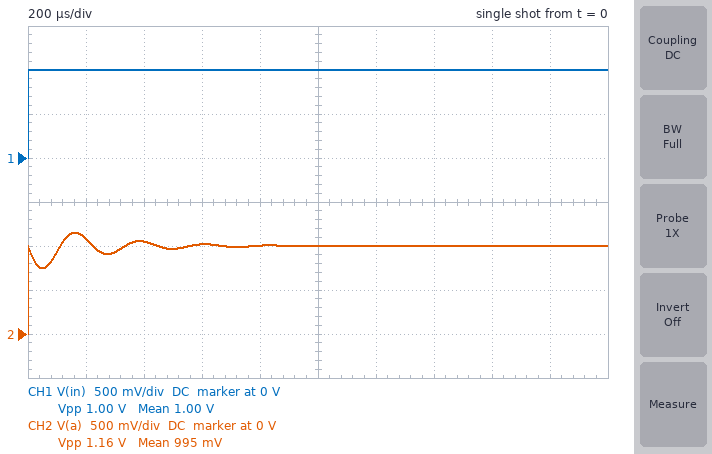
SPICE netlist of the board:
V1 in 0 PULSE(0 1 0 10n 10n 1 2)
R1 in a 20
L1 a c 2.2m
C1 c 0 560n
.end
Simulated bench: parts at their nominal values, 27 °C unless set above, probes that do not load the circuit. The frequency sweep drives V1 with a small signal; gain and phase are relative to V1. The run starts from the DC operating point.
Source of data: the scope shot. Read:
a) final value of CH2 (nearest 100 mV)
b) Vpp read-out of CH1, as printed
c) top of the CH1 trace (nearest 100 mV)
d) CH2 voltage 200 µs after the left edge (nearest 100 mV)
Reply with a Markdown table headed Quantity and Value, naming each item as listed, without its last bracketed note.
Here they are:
| Quantity | Value |
|---|---|
| final value of CH2 | 1.0 V |
| Vpp read-out of CH1, as printed | 1.00 V |
| top of the CH1 trace | 1.0 V |
| CH2 voltage 200 µs after the left edge | 1.1 V |
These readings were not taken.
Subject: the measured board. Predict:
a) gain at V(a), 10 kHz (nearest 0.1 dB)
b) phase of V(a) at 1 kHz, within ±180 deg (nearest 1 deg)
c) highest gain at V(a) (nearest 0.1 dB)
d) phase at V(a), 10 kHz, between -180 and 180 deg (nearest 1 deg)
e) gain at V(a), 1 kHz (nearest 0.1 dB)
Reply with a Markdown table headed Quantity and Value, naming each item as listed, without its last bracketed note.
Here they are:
| Quantity | Value |
|---|---|
| gain at V(a), 10 kHz | -0.1 dB |
| phase of V(a) at 1 kHz, within ±180 deg | -4 deg |
| highest gain at V(a) | 0 dB |
| phase at V(a), 10 kHz, between -180 and 180 deg | 10 deg |
| gain at V(a), 1 kHz | 0 dB |
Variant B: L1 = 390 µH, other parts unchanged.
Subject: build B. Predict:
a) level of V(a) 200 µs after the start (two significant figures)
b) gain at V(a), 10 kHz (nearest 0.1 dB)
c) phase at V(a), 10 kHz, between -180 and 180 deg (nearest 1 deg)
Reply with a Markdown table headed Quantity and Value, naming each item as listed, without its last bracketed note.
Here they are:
| Quantity | Value |
|---|---|
| level of V(a) 200 µs after the start | 1.0 V |
| gain at V(a), 10 kHz | -14.3 dB |
| phase at V(a), 10 kHz, between -180 and 180 deg | -79 deg |
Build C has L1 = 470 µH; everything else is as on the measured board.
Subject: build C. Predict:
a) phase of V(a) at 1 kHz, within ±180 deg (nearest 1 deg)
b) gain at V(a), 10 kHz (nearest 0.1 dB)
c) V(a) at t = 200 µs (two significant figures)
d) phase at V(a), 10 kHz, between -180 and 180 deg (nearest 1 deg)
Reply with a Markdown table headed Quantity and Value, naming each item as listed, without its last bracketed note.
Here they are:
| Quantity | Value |
|---|---|
| phase of V(a) at 1 kHz, within ±180 deg | -4 deg |
| gain at V(a), 10 kHz | -25.1 dB |
| V(a) at t = 200 µs | 1.0 V |
| phase at V(a), 10 kHz, between -180 and 180 deg | 87 deg |
